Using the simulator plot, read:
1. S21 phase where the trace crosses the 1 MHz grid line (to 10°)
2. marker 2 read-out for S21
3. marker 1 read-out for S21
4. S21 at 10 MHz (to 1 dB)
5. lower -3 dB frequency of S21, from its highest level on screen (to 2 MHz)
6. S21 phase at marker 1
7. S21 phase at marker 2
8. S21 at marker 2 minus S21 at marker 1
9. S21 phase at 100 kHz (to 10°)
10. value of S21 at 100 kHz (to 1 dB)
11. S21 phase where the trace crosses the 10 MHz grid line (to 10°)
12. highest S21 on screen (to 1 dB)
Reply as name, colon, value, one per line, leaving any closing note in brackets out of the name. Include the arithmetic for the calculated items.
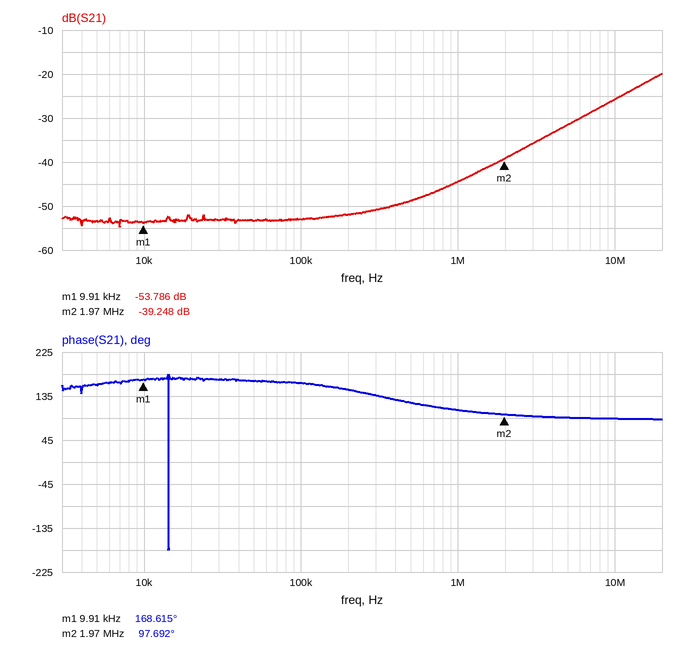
S21 phase where the trace crosses the 1 MHz grid line: 110°
marker 2 read-out for S21: -39.248 dB
marker 1 read-out for S21: -53.786 dB
S21 at 10 MHz: -26 dB
lower -3 dB frequency of S21, from its highest level on screen: 14 MHz
S21 phase at marker 1: 168.615°
S21 phase at marker 2: 97.692°
S21 at marker 2 minus S21 at marker 1: -39.248 − (-53.786) = 14.538 dB
S21 phase at 100 kHz: 160°
value of S21 at 100 kHz: -53 dB
S21 phase where the trace crosses the 10 MHz grid line: 90°
highest S21 on screen: -20 dB
